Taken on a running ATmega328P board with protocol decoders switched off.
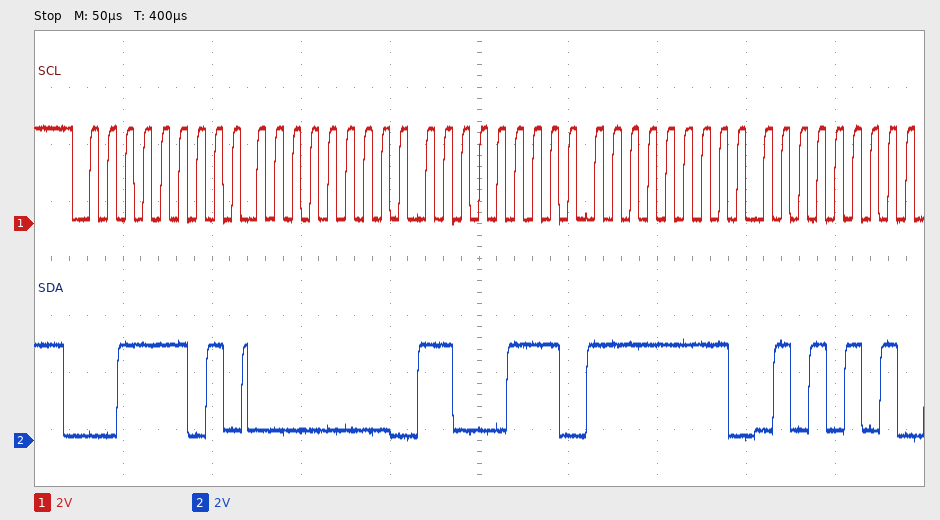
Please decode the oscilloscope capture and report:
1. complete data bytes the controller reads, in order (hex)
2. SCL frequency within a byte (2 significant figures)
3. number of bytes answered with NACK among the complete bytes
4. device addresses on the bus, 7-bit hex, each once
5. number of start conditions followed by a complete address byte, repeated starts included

00 C7 FF 55
100 kHz
0
0x1E
1
